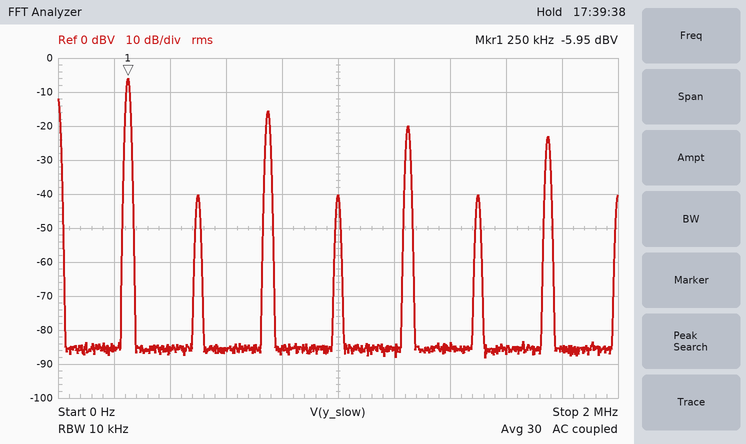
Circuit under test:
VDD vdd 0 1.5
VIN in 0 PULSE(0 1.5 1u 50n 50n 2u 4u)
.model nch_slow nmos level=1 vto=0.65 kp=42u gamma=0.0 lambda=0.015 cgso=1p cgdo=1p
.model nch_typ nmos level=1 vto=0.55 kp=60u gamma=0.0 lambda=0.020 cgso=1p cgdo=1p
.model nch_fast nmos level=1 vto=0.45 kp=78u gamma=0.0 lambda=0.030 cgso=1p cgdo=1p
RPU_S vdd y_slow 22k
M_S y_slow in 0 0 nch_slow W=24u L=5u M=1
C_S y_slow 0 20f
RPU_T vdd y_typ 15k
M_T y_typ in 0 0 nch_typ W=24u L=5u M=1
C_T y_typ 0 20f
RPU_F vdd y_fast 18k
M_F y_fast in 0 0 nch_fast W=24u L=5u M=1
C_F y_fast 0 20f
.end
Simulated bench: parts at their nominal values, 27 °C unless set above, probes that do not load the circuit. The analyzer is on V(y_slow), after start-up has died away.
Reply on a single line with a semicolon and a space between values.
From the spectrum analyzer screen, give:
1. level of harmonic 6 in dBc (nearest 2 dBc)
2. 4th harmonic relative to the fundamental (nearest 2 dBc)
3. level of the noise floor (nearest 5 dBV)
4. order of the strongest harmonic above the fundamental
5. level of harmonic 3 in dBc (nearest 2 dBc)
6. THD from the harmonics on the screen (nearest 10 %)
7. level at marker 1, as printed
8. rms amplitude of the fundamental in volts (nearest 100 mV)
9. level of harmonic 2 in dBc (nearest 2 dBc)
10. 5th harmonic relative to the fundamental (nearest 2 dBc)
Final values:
-34 dBc; -34 dBc; -85 dBV; 3; -10 dBc; 40 %; -5.95 dBV; 500 mV; -34 dBc; -14 dBc
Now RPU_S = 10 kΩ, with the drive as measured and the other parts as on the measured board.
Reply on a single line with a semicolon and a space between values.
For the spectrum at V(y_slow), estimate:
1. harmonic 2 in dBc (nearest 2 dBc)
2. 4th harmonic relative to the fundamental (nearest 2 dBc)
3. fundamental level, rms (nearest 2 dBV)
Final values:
-36 dBc; -36 dBc; -10 dBV
